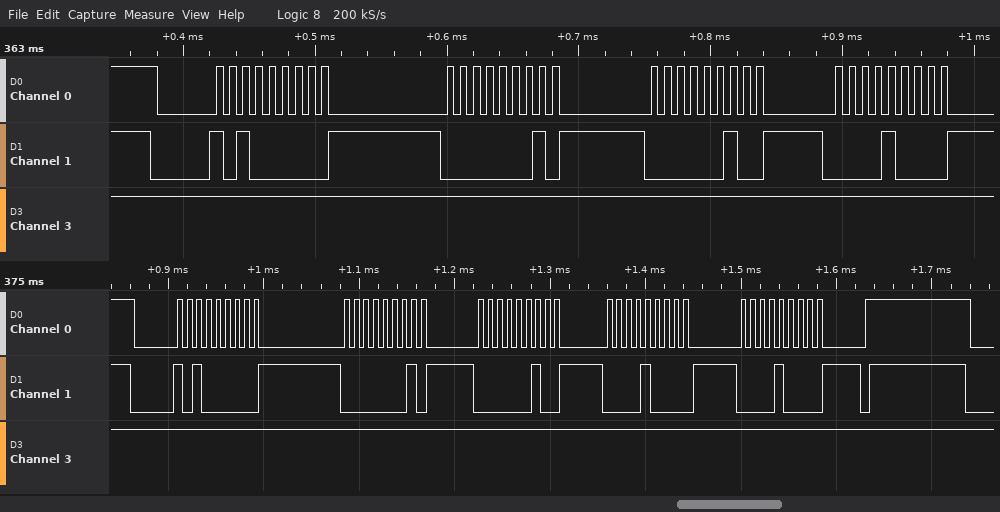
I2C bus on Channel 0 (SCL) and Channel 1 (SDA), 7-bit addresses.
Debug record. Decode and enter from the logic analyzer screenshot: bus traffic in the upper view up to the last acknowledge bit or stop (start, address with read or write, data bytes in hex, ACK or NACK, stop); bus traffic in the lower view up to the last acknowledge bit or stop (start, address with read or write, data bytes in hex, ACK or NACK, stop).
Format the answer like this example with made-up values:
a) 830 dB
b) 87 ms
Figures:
a) start, address 50 write ACK, 01 ACK, 02 ACK, 08 ACK
b) start, address 50 write ACK, 01 ACK, 02 ACK, 08 ACK, 08 ACK, stop
